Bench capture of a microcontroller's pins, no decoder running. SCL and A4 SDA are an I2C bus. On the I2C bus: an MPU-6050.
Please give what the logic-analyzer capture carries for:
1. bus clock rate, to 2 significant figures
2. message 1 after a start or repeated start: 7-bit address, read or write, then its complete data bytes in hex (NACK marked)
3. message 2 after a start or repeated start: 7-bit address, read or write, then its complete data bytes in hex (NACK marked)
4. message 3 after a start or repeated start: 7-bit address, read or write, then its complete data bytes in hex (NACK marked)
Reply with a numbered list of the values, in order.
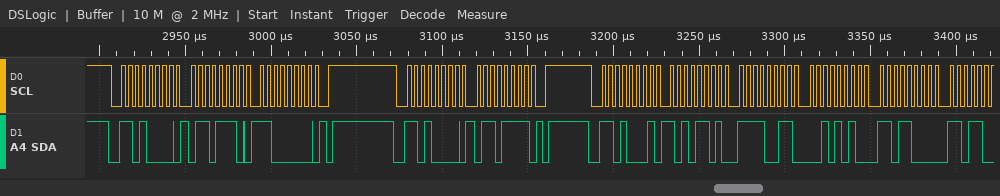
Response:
1. 250 kHz
2. 0x68 write: 6E C0
3. 0x68 write: 6F
4. 0x68 read: AD F3 2A D8
